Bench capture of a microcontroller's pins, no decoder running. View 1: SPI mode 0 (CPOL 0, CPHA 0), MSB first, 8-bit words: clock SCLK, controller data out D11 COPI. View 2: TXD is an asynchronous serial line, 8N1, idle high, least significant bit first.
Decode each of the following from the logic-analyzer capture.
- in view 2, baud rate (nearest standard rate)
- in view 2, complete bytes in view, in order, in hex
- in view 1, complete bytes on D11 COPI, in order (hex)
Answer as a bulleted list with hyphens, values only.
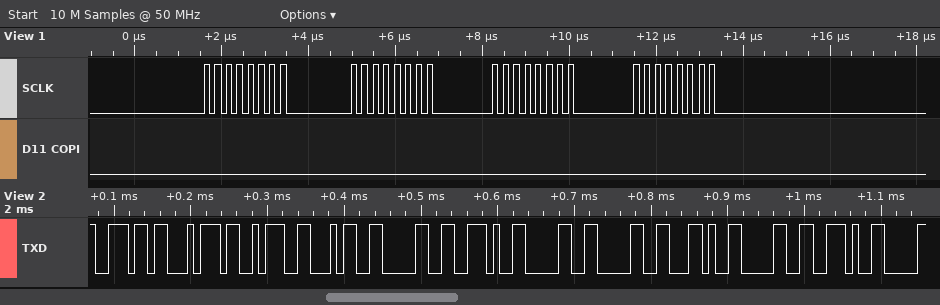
- 115200 baud
- 6E 74 3A 34 30 2E 30 30 2C 30 2E
- 00 00 00 00
